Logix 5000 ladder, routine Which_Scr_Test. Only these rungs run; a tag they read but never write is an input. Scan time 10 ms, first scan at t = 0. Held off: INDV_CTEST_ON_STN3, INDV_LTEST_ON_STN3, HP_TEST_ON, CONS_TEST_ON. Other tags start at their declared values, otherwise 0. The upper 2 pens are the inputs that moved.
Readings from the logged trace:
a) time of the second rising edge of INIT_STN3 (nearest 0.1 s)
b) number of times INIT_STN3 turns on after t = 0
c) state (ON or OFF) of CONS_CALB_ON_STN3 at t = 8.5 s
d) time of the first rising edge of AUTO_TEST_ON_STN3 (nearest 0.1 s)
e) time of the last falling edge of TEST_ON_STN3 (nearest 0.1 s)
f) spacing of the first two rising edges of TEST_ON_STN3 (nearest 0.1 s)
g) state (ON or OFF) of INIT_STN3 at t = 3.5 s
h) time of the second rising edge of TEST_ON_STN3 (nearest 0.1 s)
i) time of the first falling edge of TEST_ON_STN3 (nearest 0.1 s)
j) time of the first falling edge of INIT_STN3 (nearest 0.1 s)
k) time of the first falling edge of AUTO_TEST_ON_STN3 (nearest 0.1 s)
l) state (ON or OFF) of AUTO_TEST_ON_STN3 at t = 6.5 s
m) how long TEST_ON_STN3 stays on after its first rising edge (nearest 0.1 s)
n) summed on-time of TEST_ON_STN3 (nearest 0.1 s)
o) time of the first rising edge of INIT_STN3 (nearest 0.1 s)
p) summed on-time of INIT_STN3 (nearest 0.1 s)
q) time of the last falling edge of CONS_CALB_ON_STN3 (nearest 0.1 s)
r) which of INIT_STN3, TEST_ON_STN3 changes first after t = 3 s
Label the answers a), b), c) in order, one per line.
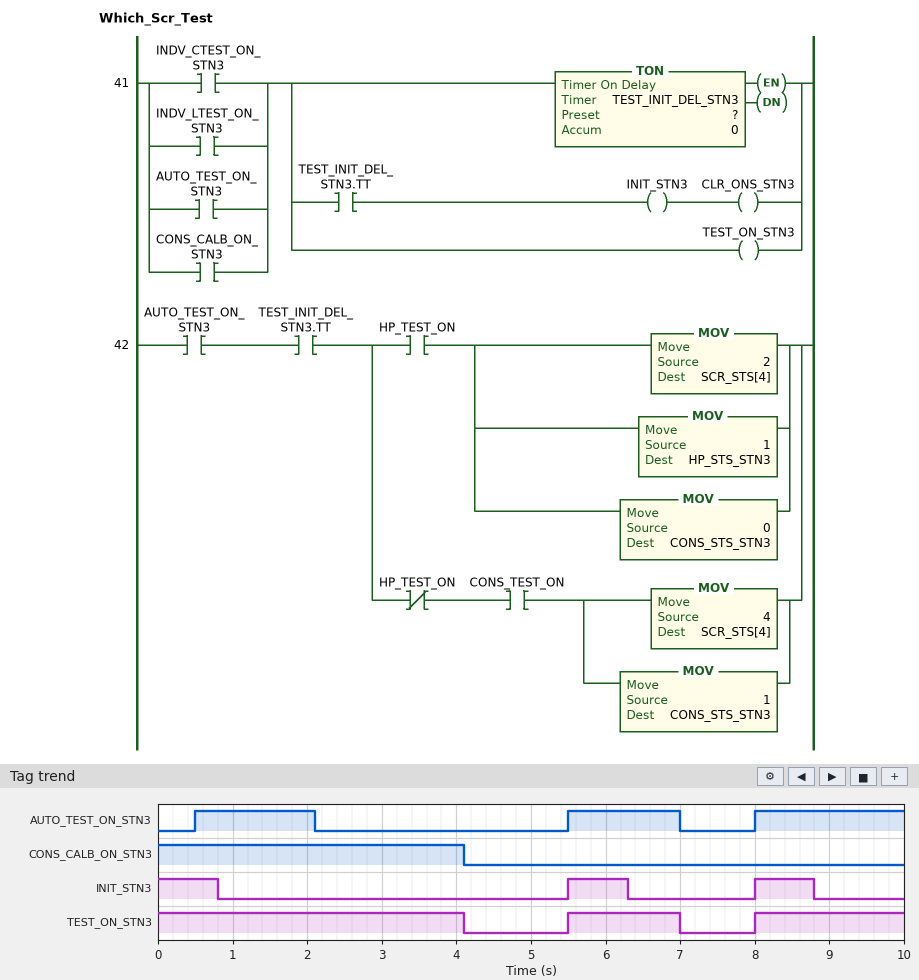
a) 8.0 s
b) 2
c) OFF
d) 0.5 s
e) 7.0 s
f) 2.5 s
g) OFF
h) 8.0 s
i) 4.1 s
j) 0.8 s
k) 2.1 s
l) ON
m) 1.5 s
n) 7.6 s
o) 5.5 s
p) 2.4 s
q) 4.1 s
r) TEST_ON_STN3
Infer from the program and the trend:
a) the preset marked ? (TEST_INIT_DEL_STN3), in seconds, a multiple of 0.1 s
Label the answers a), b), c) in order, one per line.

a) 0.8 s
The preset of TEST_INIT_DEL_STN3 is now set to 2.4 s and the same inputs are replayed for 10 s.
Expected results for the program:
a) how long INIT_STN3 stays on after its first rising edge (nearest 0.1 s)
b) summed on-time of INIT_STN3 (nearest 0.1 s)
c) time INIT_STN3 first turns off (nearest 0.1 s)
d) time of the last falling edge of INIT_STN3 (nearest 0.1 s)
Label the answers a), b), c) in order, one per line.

a) 1.5 s
b) 5.9 s
c) 2.4 s
d) 7.0 s
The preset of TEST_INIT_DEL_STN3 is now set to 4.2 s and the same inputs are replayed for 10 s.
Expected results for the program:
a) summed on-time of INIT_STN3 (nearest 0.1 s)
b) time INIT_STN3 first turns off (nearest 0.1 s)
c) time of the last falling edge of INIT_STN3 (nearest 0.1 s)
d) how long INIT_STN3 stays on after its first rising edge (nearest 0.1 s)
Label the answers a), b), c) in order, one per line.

a) 7.6 s
b) 4.1 s
c) 7.0 s
d) 1.5 s
